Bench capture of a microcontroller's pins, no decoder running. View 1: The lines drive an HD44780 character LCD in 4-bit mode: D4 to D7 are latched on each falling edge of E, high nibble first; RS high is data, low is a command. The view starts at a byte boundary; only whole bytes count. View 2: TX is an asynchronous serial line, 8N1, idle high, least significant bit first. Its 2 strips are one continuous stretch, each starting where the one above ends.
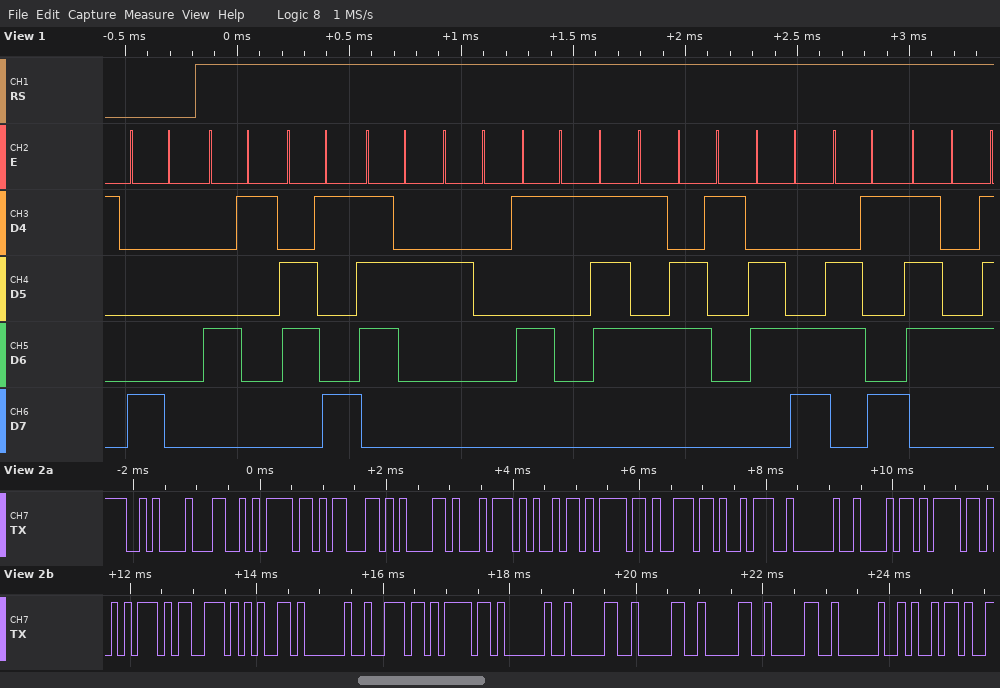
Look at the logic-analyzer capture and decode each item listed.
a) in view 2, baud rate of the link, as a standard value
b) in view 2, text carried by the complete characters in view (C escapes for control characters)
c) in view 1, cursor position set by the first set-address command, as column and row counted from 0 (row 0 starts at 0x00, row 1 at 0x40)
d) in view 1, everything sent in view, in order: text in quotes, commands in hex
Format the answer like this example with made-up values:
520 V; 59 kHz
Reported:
9600 baud; "\nLocation: house no 0000 i"; column 0, row 0; 0x80 "Air Qualit"
